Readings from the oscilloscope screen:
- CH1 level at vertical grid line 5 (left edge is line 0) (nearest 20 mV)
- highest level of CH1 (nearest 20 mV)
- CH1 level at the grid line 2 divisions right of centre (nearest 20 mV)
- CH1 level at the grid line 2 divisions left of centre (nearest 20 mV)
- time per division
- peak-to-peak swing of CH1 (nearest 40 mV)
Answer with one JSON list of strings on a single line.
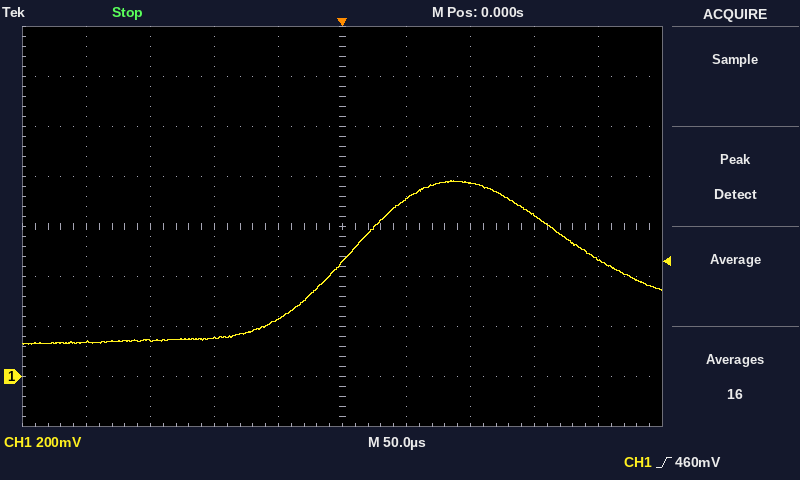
["460 mV", "780 mV", "780 mV", "160 mV", "50 µs", "640 mV"]
